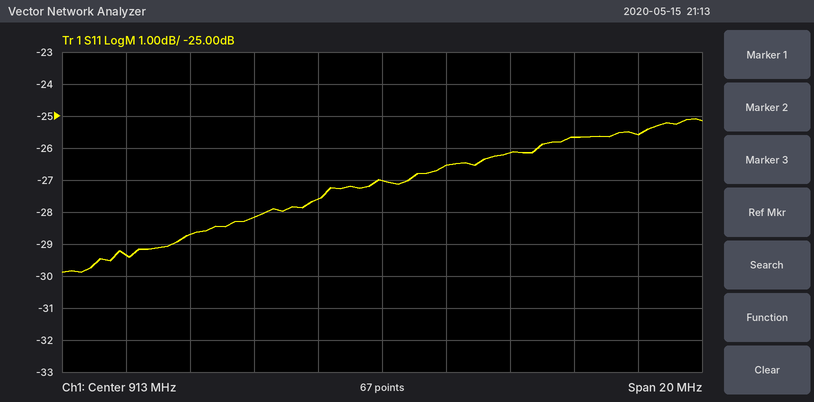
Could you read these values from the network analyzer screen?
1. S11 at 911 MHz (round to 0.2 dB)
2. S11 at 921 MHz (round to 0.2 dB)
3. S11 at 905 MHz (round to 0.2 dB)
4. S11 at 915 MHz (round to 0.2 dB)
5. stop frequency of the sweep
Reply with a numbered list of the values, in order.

1. -27.6 dB
2. -25.6 dB
3. -29.4 dB
4. -26.6 dB
5. 923 MHz
